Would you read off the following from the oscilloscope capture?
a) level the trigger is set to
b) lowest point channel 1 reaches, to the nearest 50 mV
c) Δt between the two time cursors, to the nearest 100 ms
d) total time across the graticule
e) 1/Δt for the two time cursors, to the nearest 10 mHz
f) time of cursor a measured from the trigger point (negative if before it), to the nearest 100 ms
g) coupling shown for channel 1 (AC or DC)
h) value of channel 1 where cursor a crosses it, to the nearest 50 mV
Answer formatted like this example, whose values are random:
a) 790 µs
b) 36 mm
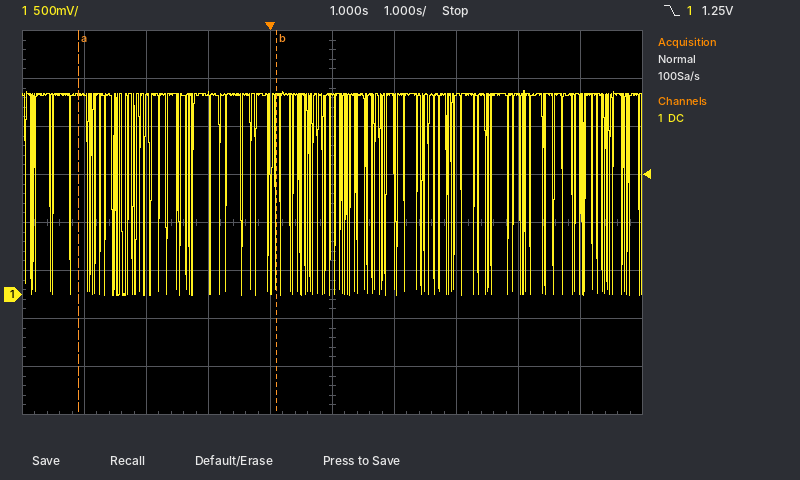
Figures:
a) 1.25 V
b) 0 mV
c) 3.2 s
d) 10 s
e) 310 mHz
f) -3.1 s
g) DC
h) 2.10 V
